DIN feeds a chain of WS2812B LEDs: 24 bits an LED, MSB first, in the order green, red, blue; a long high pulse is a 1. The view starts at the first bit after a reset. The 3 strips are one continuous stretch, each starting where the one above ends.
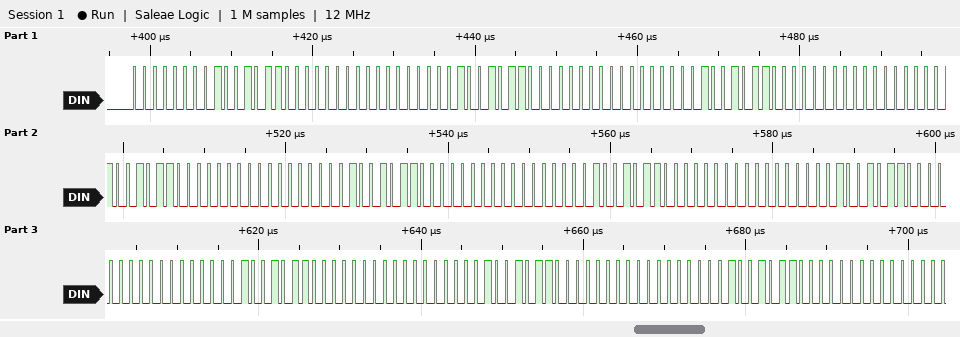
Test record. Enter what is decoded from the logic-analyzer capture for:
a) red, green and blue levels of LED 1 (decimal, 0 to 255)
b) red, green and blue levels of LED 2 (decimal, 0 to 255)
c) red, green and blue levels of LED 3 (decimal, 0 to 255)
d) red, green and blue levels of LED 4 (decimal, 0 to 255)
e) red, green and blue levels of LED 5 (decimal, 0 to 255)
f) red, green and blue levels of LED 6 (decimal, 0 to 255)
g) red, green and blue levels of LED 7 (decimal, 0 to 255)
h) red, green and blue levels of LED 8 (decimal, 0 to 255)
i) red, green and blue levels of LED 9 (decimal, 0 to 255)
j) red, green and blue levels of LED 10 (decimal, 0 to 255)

150, 0, 0
150, 0, 0
150, 0, 0
150, 0, 0
150, 0, 0
150, 0, 0
150, 0, 0
150, 0, 0
150, 0, 0
150, 0, 0
